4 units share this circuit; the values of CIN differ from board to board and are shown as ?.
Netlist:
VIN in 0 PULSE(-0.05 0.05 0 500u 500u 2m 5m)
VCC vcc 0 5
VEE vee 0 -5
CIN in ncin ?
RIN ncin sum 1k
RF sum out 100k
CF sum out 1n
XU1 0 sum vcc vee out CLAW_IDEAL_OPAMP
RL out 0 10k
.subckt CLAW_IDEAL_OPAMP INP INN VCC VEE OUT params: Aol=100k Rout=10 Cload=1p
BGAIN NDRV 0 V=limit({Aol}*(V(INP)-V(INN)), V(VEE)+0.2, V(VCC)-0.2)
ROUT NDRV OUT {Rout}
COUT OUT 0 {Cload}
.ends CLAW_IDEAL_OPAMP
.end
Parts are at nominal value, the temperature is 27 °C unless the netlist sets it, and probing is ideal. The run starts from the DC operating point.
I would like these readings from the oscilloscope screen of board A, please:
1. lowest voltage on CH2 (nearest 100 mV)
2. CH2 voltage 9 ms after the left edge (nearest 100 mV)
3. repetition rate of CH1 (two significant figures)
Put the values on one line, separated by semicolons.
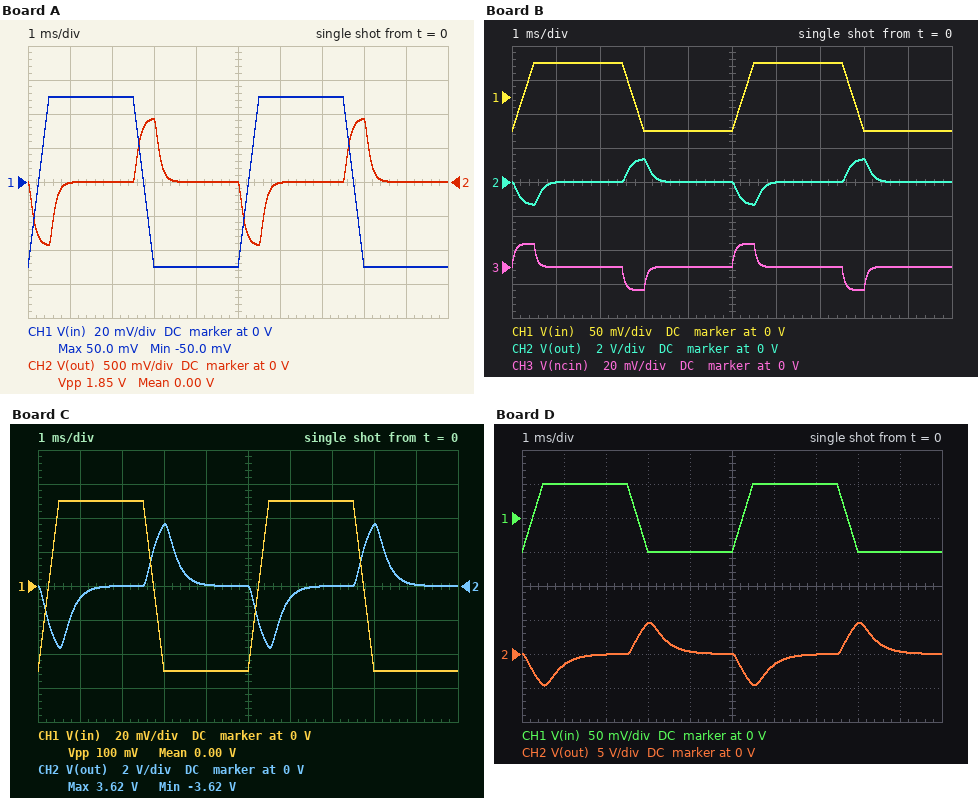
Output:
-900 mV; 0 V; 200 Hz
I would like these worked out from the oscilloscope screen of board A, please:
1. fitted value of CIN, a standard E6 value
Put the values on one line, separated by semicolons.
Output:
47 nF
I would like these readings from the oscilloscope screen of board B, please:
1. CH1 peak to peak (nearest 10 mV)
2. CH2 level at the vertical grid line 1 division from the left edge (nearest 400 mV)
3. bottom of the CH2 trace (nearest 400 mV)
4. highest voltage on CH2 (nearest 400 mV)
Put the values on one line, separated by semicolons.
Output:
100 mV; 0 V; -1.2 V; 1.2 V
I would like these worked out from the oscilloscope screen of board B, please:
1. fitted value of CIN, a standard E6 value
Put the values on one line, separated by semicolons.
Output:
68 nF
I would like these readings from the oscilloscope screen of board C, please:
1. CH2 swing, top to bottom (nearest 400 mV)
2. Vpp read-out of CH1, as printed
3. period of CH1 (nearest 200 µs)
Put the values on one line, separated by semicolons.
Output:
7.2 V; 100 mV; 5.0 ms
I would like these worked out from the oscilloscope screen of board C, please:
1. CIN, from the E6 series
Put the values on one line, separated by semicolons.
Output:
220 nF
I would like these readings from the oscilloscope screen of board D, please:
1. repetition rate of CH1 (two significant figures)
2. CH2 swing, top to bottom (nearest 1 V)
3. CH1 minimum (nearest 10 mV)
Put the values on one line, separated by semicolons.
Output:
200 Hz; 9 V; -50 mV
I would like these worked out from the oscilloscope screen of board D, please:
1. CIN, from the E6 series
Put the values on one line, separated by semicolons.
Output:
330 nF
